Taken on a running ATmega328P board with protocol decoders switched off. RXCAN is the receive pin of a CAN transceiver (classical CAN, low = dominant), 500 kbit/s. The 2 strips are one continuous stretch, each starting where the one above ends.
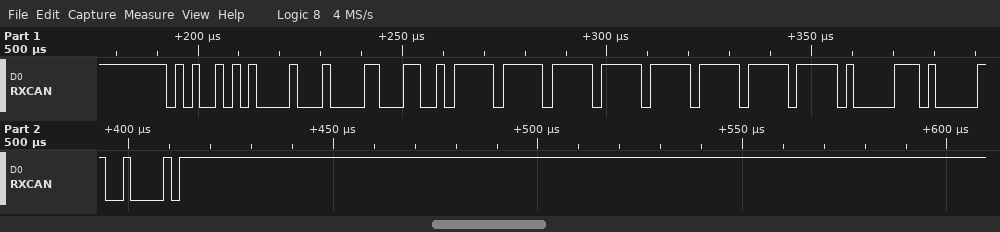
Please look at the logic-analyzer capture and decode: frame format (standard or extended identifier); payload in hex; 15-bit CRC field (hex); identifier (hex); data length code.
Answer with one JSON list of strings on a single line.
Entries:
["standard", "86 32 FF FF FF FF FF 83", "0x2090", "0x52A", "8"]
